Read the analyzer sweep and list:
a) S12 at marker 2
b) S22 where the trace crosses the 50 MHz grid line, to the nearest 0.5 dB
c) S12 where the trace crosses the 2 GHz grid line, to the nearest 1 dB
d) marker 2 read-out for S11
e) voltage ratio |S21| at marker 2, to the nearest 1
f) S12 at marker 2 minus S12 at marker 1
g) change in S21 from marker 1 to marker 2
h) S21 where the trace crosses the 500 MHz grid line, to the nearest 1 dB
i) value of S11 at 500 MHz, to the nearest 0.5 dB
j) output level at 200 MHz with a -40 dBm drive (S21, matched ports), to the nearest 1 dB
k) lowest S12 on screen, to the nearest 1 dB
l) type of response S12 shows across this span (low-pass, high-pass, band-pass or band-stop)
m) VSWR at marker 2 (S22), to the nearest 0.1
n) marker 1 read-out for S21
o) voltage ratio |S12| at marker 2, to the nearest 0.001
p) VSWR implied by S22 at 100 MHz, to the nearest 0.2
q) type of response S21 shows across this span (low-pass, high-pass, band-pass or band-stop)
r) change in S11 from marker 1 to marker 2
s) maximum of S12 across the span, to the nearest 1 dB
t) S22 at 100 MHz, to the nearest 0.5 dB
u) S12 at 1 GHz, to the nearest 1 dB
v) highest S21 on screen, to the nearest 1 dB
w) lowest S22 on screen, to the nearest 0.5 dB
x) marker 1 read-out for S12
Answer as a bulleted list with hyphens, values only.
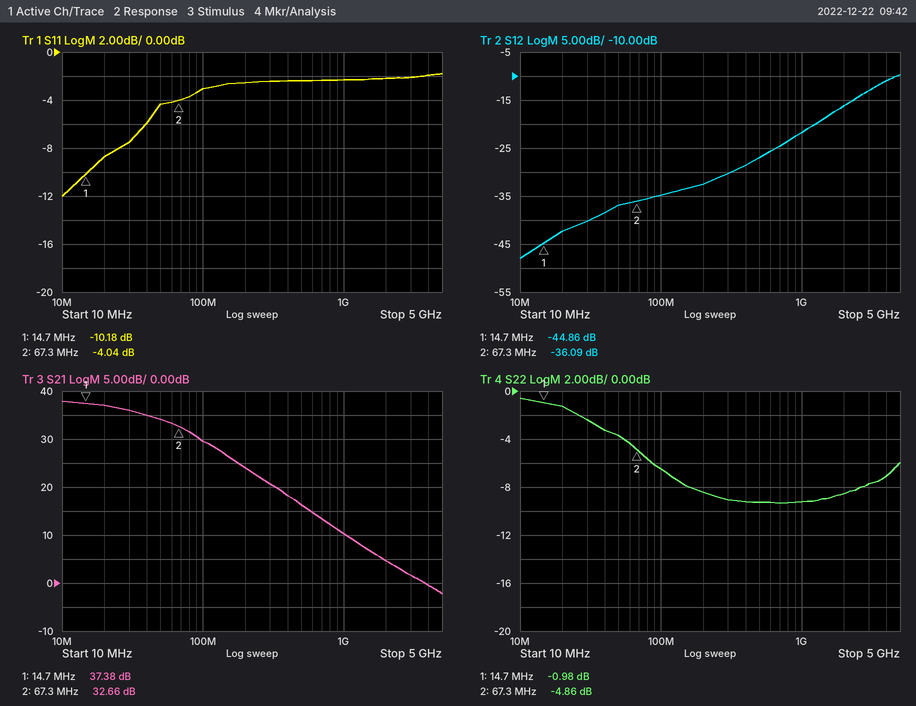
- -36.09 dB
- -3.5 dB
- -16 dB
- -4.04 dB
- 43
- 8.77 dB
- -4.72 dB
- 16 dB
- -2.5 dB
- -16 dBm
- -48 dB
- high-pass
- 3.7
- 37.38 dB
- 0.016
- 2.8
- low-pass
- 6.14 dB
- -10 dB
- -6.5 dB
- -22 dB
- 38 dB
- -9.5 dB
- -44.86 dB
